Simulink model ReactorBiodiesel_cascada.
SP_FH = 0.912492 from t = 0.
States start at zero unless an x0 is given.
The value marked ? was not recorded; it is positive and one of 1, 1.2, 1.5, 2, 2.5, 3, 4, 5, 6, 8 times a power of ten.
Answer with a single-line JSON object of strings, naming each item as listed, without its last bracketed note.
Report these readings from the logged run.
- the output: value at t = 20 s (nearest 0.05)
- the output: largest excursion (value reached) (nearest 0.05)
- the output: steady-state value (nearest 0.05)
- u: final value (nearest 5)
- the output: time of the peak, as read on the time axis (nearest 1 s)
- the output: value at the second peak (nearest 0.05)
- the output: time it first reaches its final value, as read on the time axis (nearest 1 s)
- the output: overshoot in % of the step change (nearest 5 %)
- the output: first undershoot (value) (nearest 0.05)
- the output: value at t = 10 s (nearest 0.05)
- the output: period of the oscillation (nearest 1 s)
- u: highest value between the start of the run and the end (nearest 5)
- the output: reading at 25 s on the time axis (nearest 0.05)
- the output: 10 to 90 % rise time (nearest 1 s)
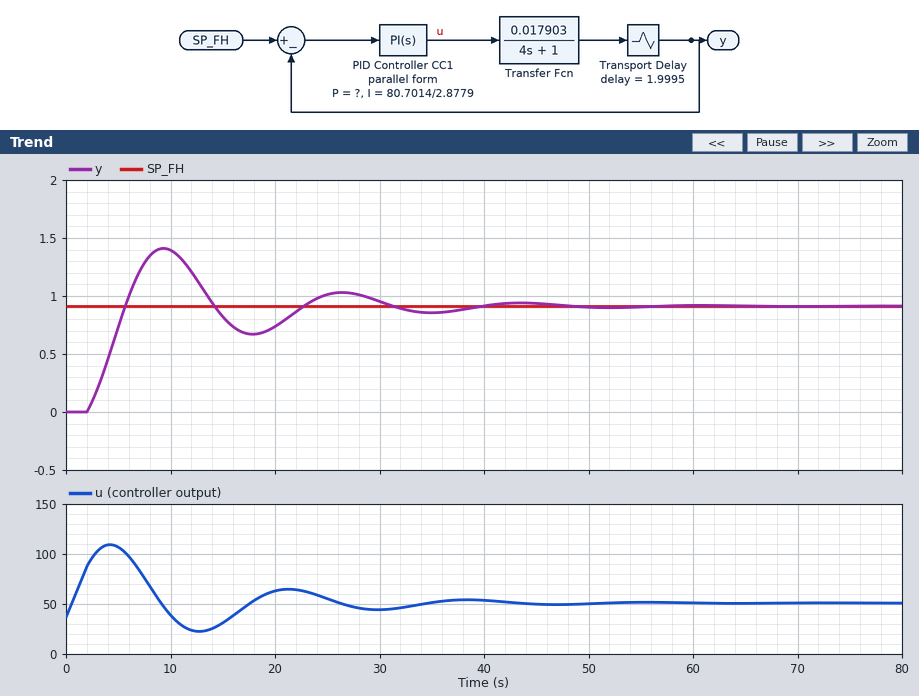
{"the output: value at t = 20 s": "0.75", "the output: largest excursion (value reached)": "1.40", "the output: steady-state value": "0.90", "u: final value": "50", "the output: time of the peak, as read on the time axis": "9 s", "the output: value at the second peak": "1.05", "the output: time it first reaches its final value, as read on the time axis": "6 s", "the output: overshoot in % of the step change": "55 %", "the output: first undershoot (value)": "0.65", "the output: value at t = 10 s": "1.40", "the output: period of the oscillation": "17 s", "u: highest value between the start of the run and the end": "110", "the output: reading at 25 s on the time axis": "1.00", "the output: 10 to 90 % rise time": "3 s"}
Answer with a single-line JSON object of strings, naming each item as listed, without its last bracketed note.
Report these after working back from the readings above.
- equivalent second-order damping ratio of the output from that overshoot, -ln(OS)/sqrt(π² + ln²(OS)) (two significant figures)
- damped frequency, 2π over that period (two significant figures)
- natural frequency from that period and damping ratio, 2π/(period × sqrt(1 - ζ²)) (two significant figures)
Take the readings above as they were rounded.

{"equivalent second-order damping ratio of the output from that overshoot, -ln(OS)/sqrt(π² + ln²(OS))": "0.19", "damped frequency, 2π over that period": "0.37 rad/s", "natural frequency from that period and damping ratio, 2π/(period × sqrt(1 - ζ²))": "0.38 rad/s"}
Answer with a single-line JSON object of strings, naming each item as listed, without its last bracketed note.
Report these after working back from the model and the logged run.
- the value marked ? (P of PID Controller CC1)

{"the value marked ?": "40"}
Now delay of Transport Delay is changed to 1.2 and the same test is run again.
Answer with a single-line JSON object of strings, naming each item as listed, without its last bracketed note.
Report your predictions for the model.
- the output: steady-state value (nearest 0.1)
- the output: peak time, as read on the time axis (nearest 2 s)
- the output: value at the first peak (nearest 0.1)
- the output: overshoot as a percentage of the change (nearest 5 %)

{"the output: steady-state value": "0.9", "the output: peak time, as read on the time axis": "8 s", "the output: value at the first peak": "1.2", "the output: overshoot as a percentage of the change": "30 %"}
